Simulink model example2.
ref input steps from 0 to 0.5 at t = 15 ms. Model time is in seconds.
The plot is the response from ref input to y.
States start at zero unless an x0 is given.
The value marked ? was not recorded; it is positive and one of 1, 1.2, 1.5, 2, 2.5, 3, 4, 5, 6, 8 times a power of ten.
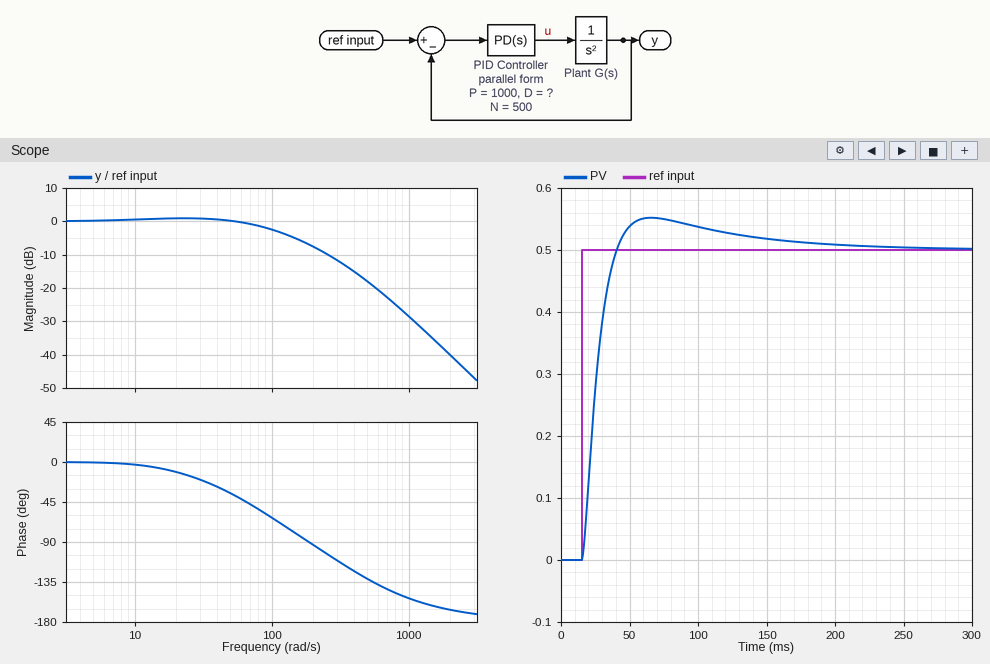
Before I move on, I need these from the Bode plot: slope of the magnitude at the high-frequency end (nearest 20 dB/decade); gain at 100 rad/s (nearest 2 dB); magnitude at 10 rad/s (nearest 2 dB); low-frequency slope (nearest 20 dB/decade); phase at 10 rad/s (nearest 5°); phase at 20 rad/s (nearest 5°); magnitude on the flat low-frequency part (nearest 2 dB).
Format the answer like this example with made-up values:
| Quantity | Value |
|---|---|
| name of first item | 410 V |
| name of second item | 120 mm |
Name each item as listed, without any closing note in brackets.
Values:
| Quantity | Value |
|---|---|
| slope of the magnitude at the high-frequency end | -40 dB/decade |
| gain at 100 rad/s | -2 dB |
| magnitude at 10 rad/s | 0 dB |
| low-frequency slope | 0 dB/decade |
| phase at 10 rad/s | -5° |
| phase at 20 rad/s | -10° |
| magnitude on the flat low-frequency part | 0 dB |
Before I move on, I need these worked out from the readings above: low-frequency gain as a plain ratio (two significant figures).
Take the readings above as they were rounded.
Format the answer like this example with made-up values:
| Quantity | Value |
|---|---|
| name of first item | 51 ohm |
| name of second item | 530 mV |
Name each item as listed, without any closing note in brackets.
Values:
| Quantity | Value |
|---|---|
| low-frequency gain as a plain ratio | 1.0 |
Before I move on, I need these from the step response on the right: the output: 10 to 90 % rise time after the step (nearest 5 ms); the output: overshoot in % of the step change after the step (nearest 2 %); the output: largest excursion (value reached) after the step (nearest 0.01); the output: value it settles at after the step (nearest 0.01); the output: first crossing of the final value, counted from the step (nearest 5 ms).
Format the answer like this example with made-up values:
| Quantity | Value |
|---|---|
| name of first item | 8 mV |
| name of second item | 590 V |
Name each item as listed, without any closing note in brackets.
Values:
| Quantity | Value |
|---|---|
| the output: 10 to 90 % rise time after the step | 15 ms |
| the output: overshoot in % of the step change after the step | 10 % |
| the output: largest excursion (value reached) after the step | 0.55 |
| the output: value it settles at after the step | 0.50 |
| the output: first crossing of the final value, counted from the step | 25 ms |
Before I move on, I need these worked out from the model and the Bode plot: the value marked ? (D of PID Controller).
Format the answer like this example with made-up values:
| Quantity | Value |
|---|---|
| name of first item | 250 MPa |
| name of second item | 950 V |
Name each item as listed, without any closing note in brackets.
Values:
| Quantity | Value |
|---|---|
| the value marked ? | 80 |
